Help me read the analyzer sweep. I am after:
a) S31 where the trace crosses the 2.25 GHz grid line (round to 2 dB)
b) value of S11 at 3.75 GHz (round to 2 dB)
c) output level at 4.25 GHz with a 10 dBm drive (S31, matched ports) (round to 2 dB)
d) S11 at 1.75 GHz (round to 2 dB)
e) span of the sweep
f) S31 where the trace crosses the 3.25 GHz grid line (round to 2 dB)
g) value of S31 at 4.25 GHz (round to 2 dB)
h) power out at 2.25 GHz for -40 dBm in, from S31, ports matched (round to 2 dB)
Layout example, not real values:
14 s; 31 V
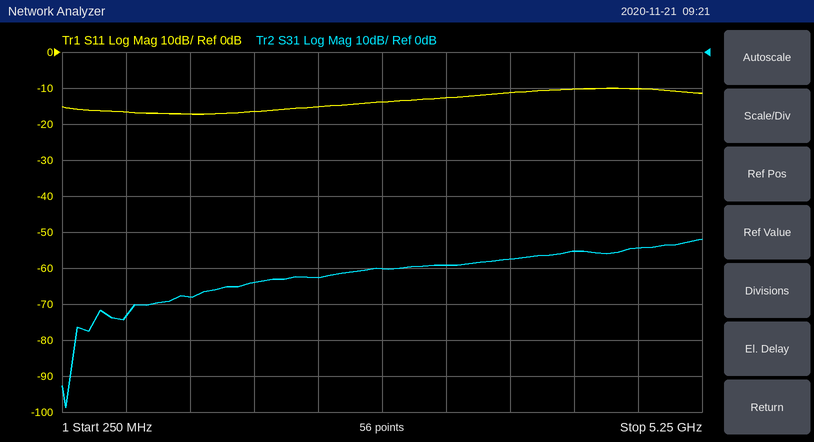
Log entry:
-62 dB; -12 dB; -46 dBm; -16 dB; 5 GHz; -60 dB; -56 dB; -102 dBm
